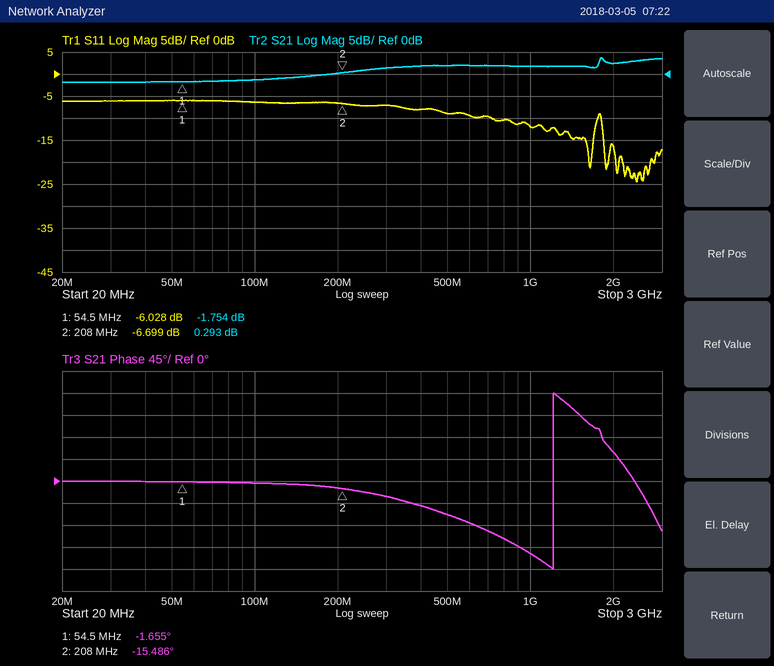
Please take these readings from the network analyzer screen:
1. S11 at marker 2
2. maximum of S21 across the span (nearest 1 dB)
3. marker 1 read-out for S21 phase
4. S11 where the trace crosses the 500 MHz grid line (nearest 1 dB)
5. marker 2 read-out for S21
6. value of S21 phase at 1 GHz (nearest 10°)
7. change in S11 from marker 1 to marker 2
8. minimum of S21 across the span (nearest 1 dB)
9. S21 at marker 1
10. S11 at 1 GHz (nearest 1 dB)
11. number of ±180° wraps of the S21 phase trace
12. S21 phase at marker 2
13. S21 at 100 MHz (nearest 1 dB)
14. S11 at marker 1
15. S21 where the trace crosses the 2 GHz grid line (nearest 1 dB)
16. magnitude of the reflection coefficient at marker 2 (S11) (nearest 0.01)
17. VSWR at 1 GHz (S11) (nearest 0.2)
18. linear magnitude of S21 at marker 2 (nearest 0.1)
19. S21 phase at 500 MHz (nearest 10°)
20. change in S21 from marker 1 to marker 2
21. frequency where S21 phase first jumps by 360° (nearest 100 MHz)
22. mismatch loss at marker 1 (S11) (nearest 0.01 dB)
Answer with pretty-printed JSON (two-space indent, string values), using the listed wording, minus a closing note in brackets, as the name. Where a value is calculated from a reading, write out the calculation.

{
  "S11 at marker 2": "-6.699 dB",
  "maximum of S21 across the span": "4 dB",
  "marker 1 read-out for S21 phase": "-1.655°",
  "S11 where the trace crosses the 500 MHz grid line": "-9 dB",
  "marker 2 read-out for S21": "0.293 dB",
  "value of S21 phase at 1 GHz": "-150°",
  "change in S11 from marker 1 to marker 2": "-6.699 − (-6.028) = -0.671 dB",
  "minimum of S21 across the span": "-2 dB",
  "S21 at marker 1": "-1.754 dB",
  "S11 at 1 GHz": "-12 dB",
  "number of ±180° wraps of the S21 phase trace": "1",
  "S21 phase at marker 2": "-15.486°",
  "S21 at 100 MHz": "-1 dB",
  "S11 at marker 1": "-6.028 dB",
  "S21 where the trace crosses the 2 GHz grid line": "2 dB",
  "magnitude of the reflection coefficient at marker 2 (S11)": "10^(-6.699/20) ≈ 0.46",
  "VSWR at 1 GHz (S11)": "|Γ| = 10^(-12/20) = 0.2512; VSWR = (1 + 0.2512)/(1 − 0.2512) ≈ 1.67, so 1.6 to the nearest 0.2",
  "linear magnitude of S21 at marker 2": "10^(0.293/20) ≈ 1.0",
  "S21 phase at 500 MHz": "-70°",
  "change in S21 from marker 1 to marker 2": "0.293 − (-1.754) = 2.047 dB",
  "frequency where S21 phase first jumps by 360°": "1.2 GHz",
  "mismatch loss at marker 1 (S11)": "−10 log10(1 − 10^(-6.028/10)) ≈ 1.25 dB"
}
